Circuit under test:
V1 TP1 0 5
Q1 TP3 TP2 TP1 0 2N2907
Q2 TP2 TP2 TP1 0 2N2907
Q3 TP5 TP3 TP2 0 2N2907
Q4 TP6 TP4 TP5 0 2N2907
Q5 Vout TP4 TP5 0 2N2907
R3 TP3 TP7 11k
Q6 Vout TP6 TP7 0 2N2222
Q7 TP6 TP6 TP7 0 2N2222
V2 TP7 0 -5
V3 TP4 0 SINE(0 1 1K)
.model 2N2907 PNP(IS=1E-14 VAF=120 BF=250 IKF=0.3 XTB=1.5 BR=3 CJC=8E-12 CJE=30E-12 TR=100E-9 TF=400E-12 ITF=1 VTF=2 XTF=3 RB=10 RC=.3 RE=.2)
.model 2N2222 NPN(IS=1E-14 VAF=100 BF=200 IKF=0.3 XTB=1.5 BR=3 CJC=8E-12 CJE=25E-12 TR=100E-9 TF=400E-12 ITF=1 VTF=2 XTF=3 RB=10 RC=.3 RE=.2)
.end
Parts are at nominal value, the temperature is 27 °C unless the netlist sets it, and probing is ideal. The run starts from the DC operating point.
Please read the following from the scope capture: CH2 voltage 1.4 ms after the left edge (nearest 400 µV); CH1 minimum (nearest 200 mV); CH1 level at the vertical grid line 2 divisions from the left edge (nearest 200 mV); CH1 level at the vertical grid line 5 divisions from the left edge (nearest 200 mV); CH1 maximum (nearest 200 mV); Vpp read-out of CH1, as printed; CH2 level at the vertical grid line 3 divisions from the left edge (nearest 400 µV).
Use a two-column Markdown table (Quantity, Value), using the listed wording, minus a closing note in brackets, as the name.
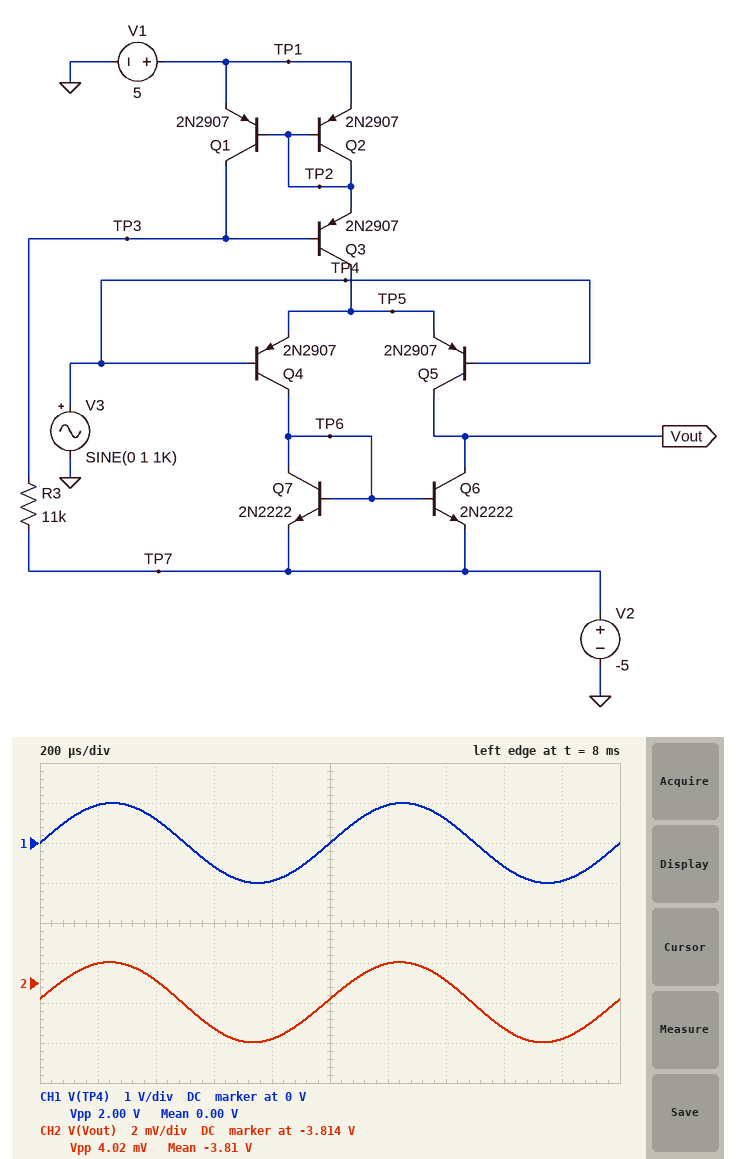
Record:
| Quantity | Value |
|---|---|
| CH2 voltage 1.4 ms after the left edge | -3.8140 V |
| CH1 minimum | -1.0 V |
| CH1 level at the vertical grid line 2 divisions from the left edge | 600 mV |
| CH1 level at the vertical grid line 5 divisions from the left edge | 0 V |
| CH1 maximum | 1.0 V |
| Vpp read-out of CH1, as printed | 2.00 V |
| CH2 level at the vertical grid line 3 divisions from the left edge | -3.8164 V |
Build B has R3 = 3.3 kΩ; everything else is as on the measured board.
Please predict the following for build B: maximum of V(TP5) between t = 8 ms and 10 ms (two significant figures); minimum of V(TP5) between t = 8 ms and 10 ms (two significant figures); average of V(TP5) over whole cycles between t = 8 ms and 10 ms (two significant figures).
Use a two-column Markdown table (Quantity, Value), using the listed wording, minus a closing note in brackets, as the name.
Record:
| Quantity | Value |
|---|---|
| maximum of V(TP5) between t = 8 ms and 10 ms | 1.7 V |
| minimum of V(TP5) between t = 8 ms and 10 ms | -340 mV |
| average of V(TP5) over whole cycles between t = 8 ms and 10 ms | 660 mV |
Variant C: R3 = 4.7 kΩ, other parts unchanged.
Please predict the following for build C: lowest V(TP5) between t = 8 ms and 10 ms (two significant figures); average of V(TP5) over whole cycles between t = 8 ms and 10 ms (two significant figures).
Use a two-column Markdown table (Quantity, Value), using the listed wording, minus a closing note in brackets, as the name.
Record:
| Quantity | Value |
|---|---|
| lowest V(TP5) between t = 8 ms and 10 ms | -350 mV |
| average of V(TP5) over whole cycles between t = 8 ms and 10 ms | 650 mV |
